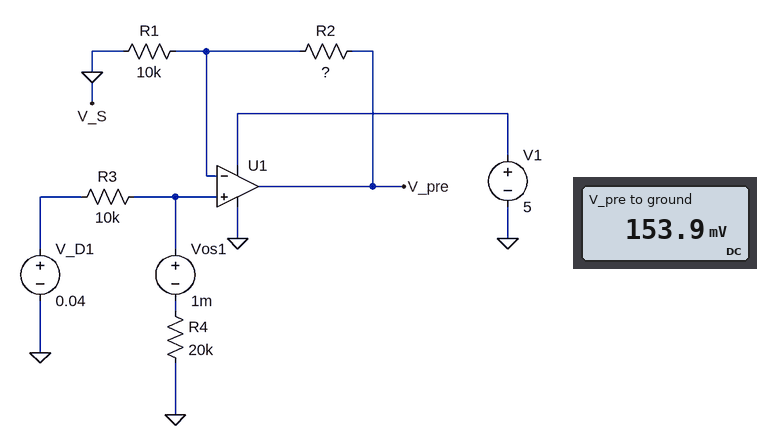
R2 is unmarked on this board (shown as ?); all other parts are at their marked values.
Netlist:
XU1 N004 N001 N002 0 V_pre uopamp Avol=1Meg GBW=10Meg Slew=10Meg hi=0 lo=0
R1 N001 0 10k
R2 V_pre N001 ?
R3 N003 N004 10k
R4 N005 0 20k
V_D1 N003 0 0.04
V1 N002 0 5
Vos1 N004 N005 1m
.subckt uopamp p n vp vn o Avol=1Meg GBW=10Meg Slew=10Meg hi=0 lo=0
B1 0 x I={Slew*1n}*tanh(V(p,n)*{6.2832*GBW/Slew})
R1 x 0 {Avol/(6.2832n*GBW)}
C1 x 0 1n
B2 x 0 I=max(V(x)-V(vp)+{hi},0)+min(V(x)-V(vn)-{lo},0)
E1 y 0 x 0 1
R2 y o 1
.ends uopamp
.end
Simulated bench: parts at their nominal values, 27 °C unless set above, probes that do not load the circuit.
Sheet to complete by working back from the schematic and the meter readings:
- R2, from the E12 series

47 kΩ
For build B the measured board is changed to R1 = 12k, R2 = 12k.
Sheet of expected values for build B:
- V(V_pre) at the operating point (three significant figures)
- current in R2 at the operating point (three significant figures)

54.0 mV
2.25 µA
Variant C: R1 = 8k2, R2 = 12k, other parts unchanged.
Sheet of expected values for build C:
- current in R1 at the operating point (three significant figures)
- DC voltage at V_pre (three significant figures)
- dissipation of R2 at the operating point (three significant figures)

3.29 µA
66.5 mV
130 nW
